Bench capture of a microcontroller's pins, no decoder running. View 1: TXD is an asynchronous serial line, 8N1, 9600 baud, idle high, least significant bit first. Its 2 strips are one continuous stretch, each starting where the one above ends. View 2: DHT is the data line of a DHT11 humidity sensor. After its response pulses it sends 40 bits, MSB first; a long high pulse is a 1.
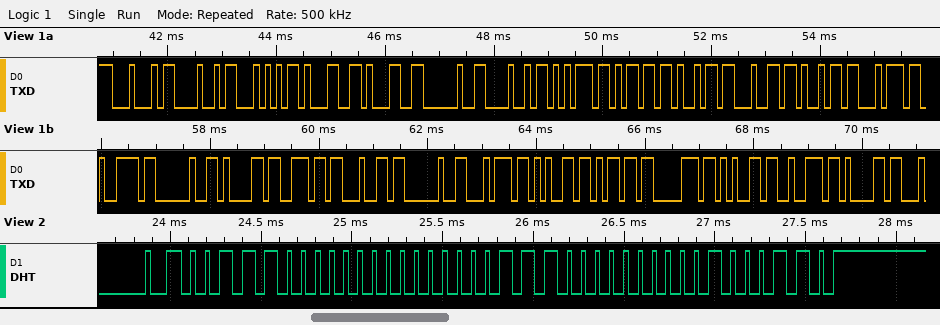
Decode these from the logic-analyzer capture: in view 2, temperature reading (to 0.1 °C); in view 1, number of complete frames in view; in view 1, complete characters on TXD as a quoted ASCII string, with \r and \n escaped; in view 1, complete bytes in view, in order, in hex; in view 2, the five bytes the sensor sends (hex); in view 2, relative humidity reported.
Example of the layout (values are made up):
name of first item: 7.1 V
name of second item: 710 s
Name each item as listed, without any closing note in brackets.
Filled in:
in view 2, temperature reading: 14.0 °C
in view 1, number of complete frames in view: 26
in view 1, complete characters on TXD as a quoted ASCII string, with \r and \n escaped: "DHT11 Humidity and tempera"
in view 1, complete bytes in view, in order, in hex: 44 48 54 31 31 20 48 75 6D 69 64 69 74 79 20 61 6E 64 20 74 65 6D 70 65 72 61
in view 2, the five bytes the sensor sends: 38 00 0E 00 46
in view 2, relative humidity reported: 56 %
